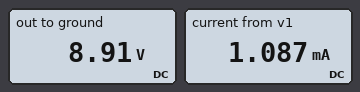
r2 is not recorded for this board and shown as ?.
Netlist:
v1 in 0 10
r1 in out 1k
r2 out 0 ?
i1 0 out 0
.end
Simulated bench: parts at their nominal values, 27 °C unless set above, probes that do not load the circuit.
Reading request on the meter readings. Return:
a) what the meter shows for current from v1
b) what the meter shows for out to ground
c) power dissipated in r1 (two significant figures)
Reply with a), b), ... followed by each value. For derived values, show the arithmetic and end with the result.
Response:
a) 1.087 mA
b) 8.91 V
c) (10 V - 8.91 V)^2 / 1 kΩ = 1.2 mW
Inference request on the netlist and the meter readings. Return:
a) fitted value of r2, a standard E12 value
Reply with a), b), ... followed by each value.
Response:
a) 8.2 kΩ
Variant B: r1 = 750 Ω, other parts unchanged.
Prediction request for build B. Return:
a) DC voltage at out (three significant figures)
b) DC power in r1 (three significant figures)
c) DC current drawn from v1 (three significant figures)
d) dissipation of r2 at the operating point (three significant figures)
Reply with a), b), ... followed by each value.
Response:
a) 9.16 V
b) 936 µW
c) 1.12 mA
d) 10.2 mW
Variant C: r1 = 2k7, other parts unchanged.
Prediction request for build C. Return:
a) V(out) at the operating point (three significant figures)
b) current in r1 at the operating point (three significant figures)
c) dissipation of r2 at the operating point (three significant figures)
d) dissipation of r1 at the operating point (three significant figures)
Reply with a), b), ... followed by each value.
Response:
a) 7.52 V
b) 917 µA
c) 6.90 mW
d) 2.27 mW
